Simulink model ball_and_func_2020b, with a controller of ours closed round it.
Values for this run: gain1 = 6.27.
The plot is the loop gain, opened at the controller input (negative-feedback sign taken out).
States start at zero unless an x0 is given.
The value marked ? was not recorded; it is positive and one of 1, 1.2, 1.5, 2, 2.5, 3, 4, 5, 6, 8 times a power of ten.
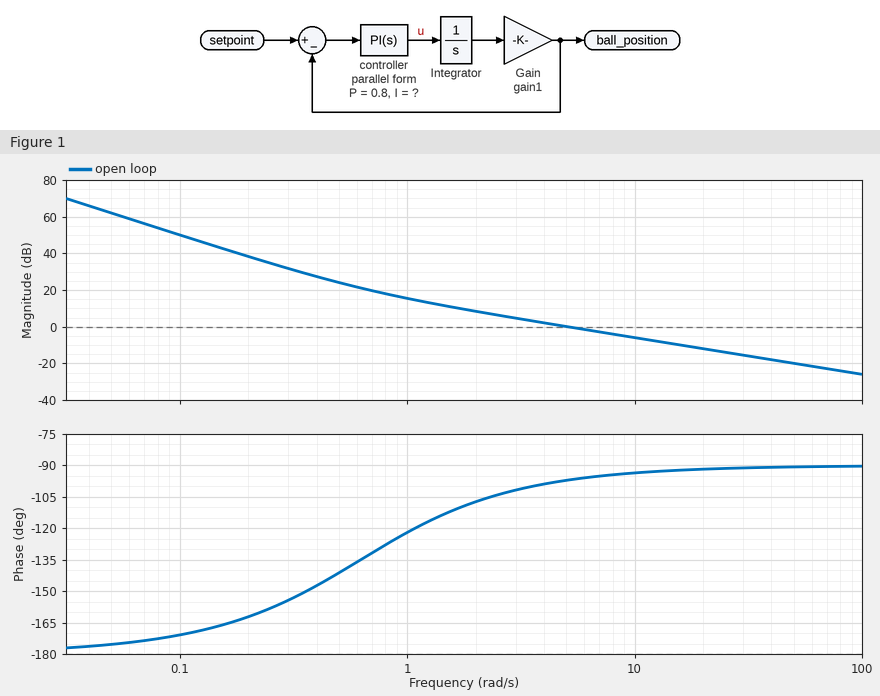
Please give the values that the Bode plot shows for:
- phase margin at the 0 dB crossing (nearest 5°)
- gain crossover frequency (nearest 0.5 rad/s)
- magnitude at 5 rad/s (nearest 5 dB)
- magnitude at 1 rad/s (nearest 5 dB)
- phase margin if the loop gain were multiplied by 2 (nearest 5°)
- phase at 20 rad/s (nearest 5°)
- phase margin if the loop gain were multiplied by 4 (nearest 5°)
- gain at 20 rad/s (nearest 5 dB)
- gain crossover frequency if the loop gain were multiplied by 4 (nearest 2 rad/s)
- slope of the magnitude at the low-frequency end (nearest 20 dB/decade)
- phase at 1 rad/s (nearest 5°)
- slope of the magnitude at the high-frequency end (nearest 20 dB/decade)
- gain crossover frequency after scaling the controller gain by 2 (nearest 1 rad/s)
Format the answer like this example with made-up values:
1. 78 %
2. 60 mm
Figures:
1. 85°
2. 5.0 rad/s
3. 0 dB
4. 15 dB
5. 85°
6. -90°
7. 90°
8. -10 dB
9. 20 rad/s
10. -40 dB/decade
11. -120°
12. -20 dB/decade
13. 10 rad/s
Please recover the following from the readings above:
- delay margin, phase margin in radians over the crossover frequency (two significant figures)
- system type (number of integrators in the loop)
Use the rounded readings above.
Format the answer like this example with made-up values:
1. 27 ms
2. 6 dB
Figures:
1. 0.30 s
2. 2
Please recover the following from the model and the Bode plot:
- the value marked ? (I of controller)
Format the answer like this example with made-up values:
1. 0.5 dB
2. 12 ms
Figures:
1. 0.5
